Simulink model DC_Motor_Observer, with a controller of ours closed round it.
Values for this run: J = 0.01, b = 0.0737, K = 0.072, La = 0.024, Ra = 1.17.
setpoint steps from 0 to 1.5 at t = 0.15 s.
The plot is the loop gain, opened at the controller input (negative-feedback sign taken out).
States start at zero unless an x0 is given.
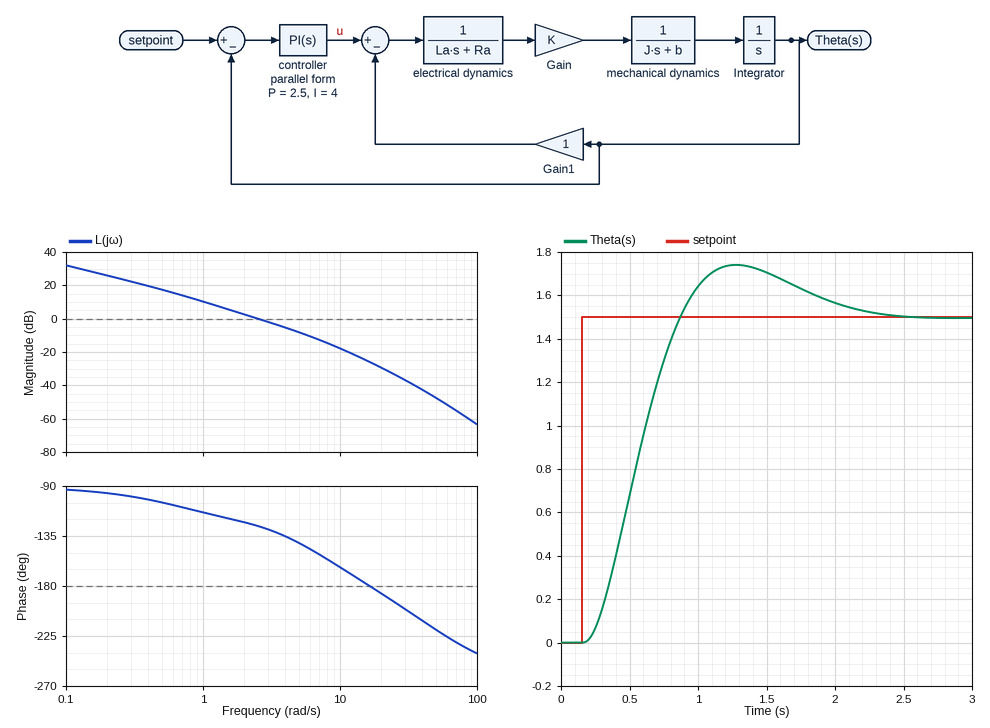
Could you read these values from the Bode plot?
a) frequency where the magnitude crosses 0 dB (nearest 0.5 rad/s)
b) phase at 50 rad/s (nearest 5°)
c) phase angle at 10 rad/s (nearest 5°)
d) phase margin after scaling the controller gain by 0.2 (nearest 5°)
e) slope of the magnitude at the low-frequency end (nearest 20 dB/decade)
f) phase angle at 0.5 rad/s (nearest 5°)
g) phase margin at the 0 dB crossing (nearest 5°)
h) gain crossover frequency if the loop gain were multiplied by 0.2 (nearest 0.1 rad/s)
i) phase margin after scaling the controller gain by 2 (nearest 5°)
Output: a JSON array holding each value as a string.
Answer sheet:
["2.5 rad/s", "-220°", "-165°", "70°", "-20 dB/decade", "-105°", "55°", "0.7 rad/s", "45°"]
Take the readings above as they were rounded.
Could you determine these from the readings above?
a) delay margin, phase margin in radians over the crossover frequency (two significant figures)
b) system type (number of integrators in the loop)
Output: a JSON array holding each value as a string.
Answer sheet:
["0.38 s", "1"]
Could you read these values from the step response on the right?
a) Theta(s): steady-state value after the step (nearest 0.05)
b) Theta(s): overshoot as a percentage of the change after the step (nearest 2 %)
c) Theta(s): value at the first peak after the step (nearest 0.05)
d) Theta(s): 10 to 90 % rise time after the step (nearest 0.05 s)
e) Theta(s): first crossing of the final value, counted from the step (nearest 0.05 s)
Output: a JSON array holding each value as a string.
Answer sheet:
["1.50", "16 %", "1.75", "0.50 s", "0.70 s"]
